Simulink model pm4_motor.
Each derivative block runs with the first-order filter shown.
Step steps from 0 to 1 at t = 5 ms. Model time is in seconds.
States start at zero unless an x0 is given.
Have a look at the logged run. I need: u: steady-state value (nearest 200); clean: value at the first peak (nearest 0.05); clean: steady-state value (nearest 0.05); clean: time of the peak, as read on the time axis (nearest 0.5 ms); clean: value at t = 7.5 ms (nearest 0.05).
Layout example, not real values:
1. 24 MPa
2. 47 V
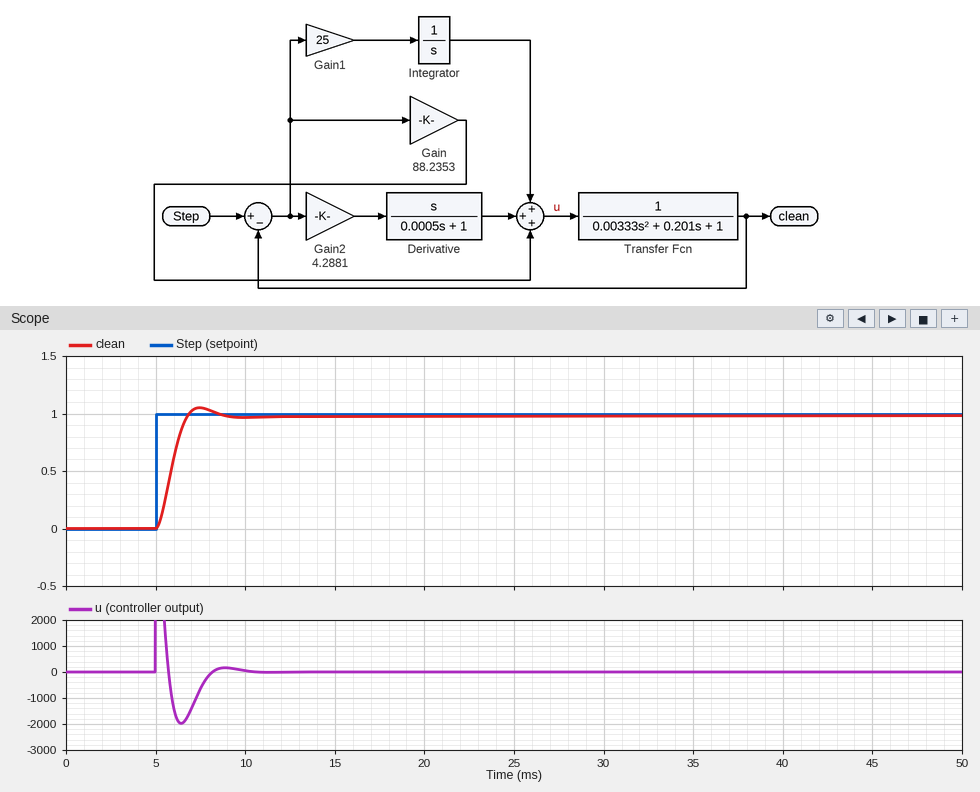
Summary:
1. 0
2. 1.05
3. 1.00
4. 7.5 ms
5. 1.05
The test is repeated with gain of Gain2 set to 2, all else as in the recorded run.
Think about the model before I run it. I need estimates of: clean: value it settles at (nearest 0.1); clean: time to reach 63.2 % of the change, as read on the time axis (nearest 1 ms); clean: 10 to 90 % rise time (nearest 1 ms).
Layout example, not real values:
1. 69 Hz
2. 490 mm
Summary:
1. 1.0
2. 7 ms
3. 3 ms
